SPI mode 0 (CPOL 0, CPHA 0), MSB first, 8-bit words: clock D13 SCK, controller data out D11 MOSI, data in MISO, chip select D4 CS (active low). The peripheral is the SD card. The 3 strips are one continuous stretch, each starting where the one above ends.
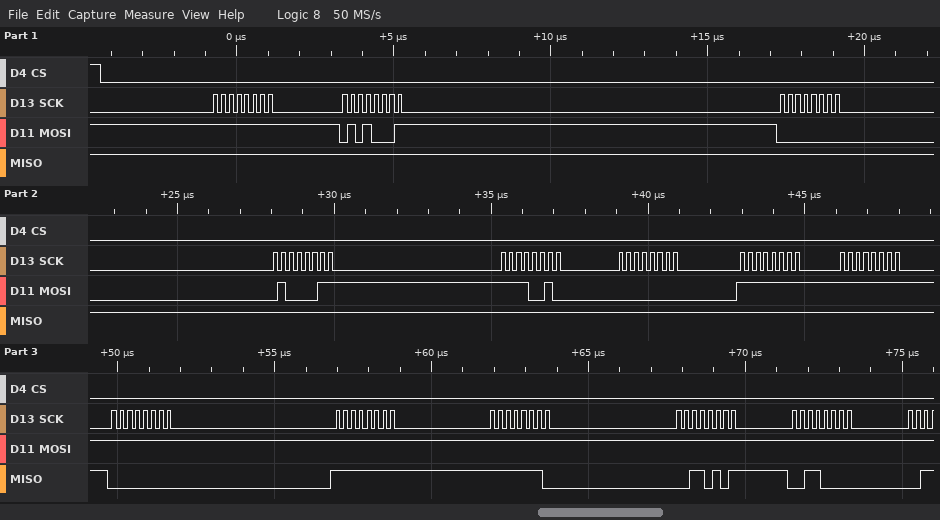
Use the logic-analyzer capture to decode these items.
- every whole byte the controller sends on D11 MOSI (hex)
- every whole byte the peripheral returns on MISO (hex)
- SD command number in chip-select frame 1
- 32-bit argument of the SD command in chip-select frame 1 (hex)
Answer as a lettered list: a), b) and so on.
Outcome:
a) FF 51 00 43 F2 00 FF FF FF FF FF FF FF
b) FF FF FF FF FF FF FF FF 00 FF FE 35 30
c) CMD17
d) 0x0043F200
